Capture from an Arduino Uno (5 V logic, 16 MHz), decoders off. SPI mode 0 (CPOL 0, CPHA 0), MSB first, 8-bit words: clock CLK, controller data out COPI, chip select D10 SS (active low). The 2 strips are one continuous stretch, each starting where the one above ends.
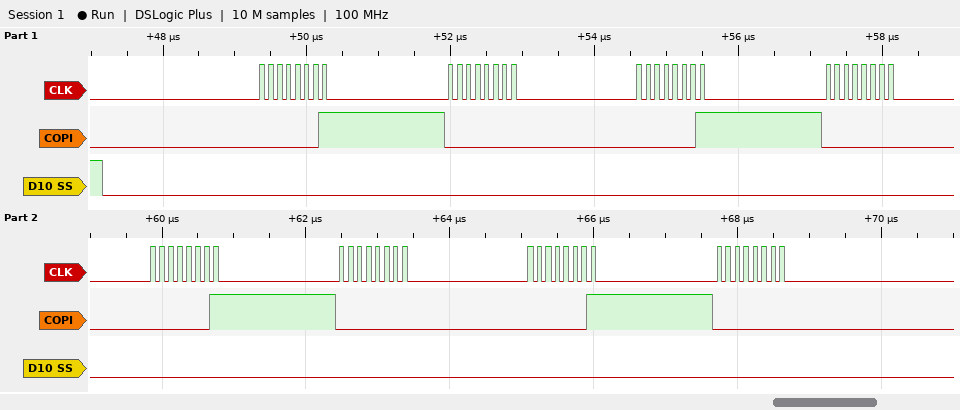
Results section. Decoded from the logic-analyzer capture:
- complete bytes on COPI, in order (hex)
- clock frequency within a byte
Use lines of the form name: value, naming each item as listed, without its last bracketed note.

complete bytes on COPI, in order: 01 00 01 00 01 00 01 00
clock frequency within a byte: 8 MHz
